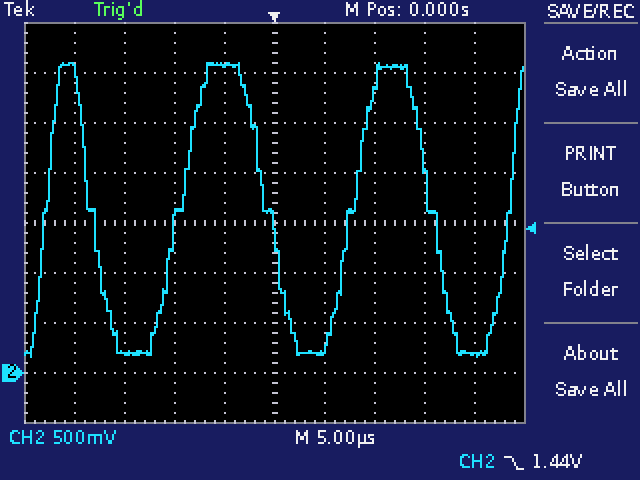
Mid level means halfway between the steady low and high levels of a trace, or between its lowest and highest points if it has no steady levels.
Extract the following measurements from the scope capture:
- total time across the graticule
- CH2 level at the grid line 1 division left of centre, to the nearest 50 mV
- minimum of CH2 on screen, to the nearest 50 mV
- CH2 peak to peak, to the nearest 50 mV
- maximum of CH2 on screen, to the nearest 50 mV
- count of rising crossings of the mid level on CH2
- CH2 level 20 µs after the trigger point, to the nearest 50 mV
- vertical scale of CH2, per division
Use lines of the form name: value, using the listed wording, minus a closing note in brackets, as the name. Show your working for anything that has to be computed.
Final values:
total time across the graticule: 50 µs
CH2 level at the grid line 1 division left of centre, to the nearest 50 mV: 3.10 V
minimum of CH2 on screen, to the nearest 50 mV: 150 mV
CH2 peak to peak, to the nearest 50 mV: 3.10 V − (150 mV) = 2.95 V
maximum of CH2 on screen, to the nearest 50 mV: 3.10 V
count of rising crossings of the mid level on CH2: 4
CH2 level 20 µs after the trigger point, to the nearest 50 mV: 200 mV
vertical scale of CH2, per division: 500 mV
